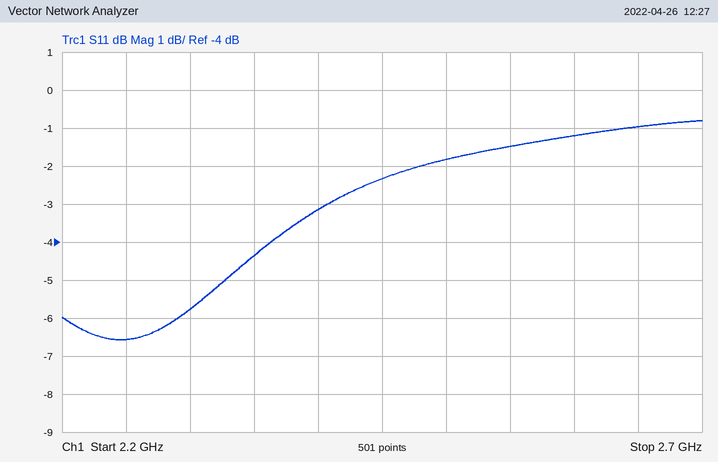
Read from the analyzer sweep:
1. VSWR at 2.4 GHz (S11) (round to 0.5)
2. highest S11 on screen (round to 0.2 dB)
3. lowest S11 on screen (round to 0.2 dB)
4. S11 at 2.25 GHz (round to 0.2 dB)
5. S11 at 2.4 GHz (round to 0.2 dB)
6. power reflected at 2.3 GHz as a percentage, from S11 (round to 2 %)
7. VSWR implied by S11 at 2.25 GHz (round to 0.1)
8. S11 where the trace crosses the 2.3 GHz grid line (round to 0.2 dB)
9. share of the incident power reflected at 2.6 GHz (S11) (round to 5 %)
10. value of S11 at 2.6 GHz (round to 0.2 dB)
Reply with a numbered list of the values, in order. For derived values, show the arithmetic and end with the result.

1. |Γ| = 10^(-3.2/20) = 0.6918; VSWR = (1 + 0.6918)/(1 − 0.6918) ≈ 5.5
2. -0.8 dB
3. -6.6 dB
4. -6.6 dB
5. -3.2 dB
6. 10^(-5.8/10) ≈ 26 %
7. |Γ| = 10^(-6.6/20) = 0.4677; VSWR = (1 + 0.4677)/(1 − 0.4677) ≈ 2.8
8. -5.8 dB
9. 10^(-1.2/10) ≈ 75.9 %, so 75 % to the nearest 5 %
10. -1.2 dB
